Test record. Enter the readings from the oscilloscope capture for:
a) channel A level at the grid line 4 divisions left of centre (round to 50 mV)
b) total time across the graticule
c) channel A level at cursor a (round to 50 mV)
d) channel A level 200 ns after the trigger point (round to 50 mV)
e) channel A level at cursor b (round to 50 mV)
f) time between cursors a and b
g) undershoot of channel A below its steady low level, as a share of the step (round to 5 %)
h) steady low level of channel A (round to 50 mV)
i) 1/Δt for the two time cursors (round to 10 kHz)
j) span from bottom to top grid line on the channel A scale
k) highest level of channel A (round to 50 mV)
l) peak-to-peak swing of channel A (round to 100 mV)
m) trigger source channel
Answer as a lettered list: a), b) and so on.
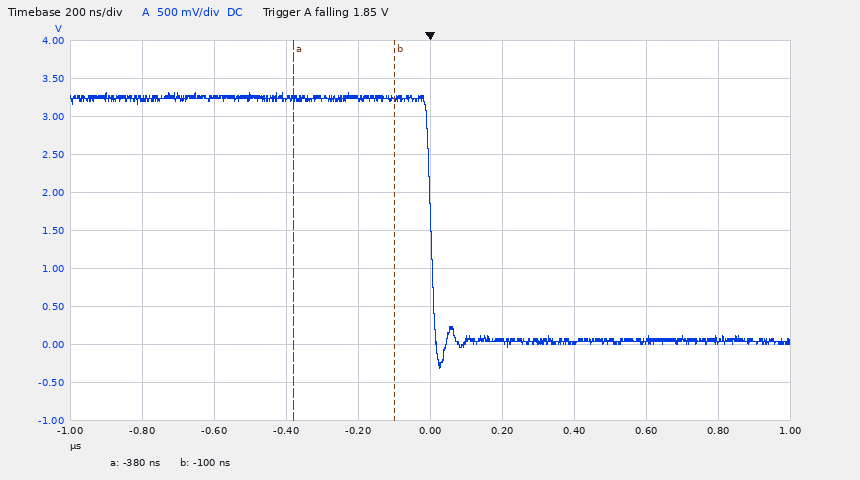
a) 3.25 V
b) 2 µs
c) 3.25 V
d) 50 mV
e) 3.25 V
f) 280 ns
g) 10 %
h) 50 mV
i) 3.57 MHz
j) 5 V
k) 3.30 V
l) 3.60 V
m) channel A
